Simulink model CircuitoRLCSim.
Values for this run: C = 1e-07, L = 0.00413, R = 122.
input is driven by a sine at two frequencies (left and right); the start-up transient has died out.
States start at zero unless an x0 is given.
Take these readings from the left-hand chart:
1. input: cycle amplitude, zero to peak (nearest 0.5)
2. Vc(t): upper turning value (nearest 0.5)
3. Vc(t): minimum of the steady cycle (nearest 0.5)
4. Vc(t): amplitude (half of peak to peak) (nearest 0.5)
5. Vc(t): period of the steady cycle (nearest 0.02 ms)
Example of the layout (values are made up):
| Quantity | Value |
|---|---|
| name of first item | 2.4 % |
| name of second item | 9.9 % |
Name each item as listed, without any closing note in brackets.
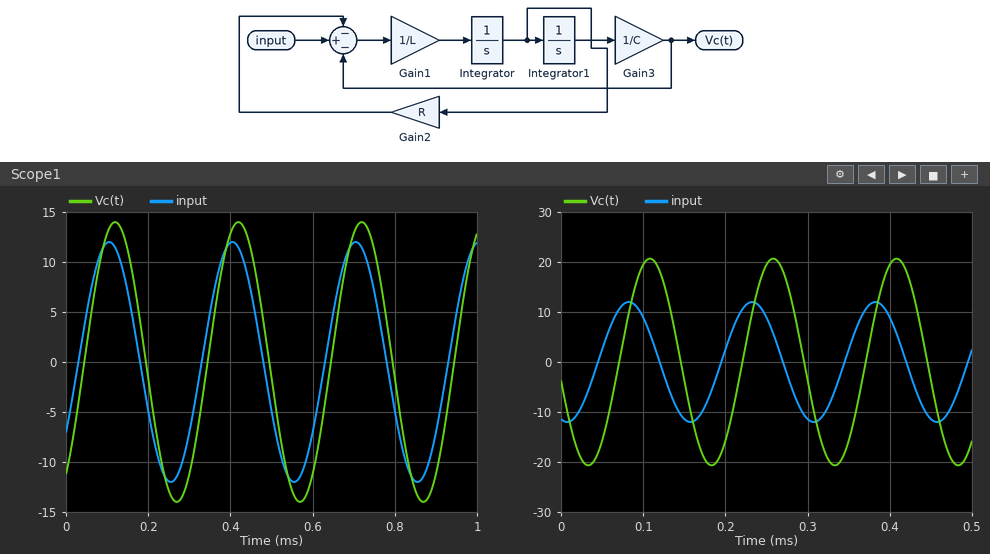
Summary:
| Quantity | Value |
|---|---|
| input: cycle amplitude, zero to peak | 12.0 |
| Vc(t): upper turning value | 14.0 |
| Vc(t): minimum of the steady cycle | -14.0 |
| Vc(t): amplitude (half of peak to peak) | 14.0 |
| Vc(t): period of the steady cycle | 0.30 ms |
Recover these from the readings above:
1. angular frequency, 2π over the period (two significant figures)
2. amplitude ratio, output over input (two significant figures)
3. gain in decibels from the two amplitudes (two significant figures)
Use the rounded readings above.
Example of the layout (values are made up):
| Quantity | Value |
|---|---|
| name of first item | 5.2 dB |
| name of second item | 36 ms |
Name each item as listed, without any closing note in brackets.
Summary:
| Quantity | Value |
|---|---|
| angular frequency, 2π over the period | 21 rad/ms |
| amplitude ratio, output over input | 1.2 |
| gain in decibels from the two amplitudes | 1.3 dB |
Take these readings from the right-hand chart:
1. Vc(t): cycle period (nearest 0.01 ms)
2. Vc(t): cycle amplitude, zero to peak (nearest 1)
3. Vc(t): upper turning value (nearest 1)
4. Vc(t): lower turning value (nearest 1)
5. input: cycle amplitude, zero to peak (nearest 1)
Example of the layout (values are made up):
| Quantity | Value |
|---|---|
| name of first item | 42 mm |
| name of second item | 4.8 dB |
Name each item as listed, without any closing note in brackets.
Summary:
| Quantity | Value |
|---|---|
| Vc(t): cycle period | 0.15 ms |
| Vc(t): cycle amplitude, zero to peak | 21 |
| Vc(t): upper turning value | 21 |
| Vc(t): lower turning value | -21 |
| input: cycle amplitude, zero to peak | 12 |
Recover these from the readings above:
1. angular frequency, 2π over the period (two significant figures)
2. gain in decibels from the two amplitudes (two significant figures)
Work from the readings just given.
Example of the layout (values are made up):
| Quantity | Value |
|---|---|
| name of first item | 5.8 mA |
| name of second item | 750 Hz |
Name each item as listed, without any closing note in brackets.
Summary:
| Quantity | Value |
|---|---|
| angular frequency, 2π over the period | 42 rad/ms |
| gain in decibels from the two amplitudes | 4.9 dB |
